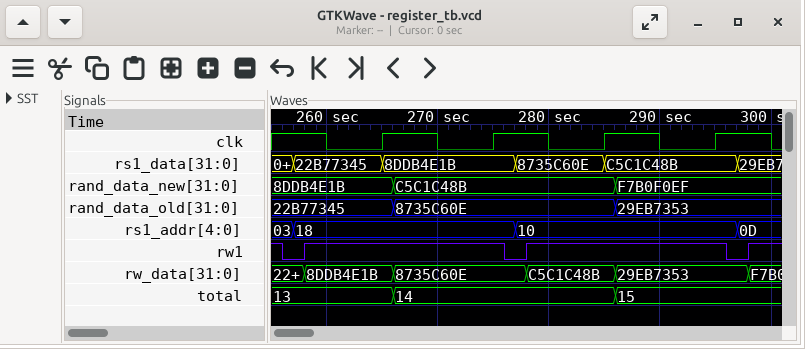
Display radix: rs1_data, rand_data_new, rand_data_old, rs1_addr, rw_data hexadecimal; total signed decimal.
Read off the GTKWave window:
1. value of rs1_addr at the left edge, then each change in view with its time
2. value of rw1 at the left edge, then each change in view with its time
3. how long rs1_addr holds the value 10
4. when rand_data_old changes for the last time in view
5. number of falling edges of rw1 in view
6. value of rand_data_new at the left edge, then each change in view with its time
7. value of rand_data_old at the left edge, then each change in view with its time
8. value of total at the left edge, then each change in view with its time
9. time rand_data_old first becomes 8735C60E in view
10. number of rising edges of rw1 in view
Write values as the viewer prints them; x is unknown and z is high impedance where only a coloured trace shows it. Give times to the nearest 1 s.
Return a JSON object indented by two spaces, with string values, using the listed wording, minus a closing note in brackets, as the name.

{
  "value of rs1_addr at the left edge, then each change in view with its time": "03, 18 at 257 s, 10 at 277 s, 0D at 297 s",
  "value of rw1 at the left edge, then each change in view with its time": "1, 0 at 256 s, 1 at 258 s, 0 at 276 s, 1 at 278 s, 0 at 296 s, 1 at 298 s",
  "how long rs1_addr holds the value 10": "20 s",
  "when rand_data_old changes for the last time in view": "286 s",
  "number of falling edges of rw1 in view": "3",
  "value of rand_data_new at the left edge, then each change in view with its time": "8DDB4E1B, C5C1C48B at 266 s, F7B0F0EF at 286 s",
  "value of rand_data_old at the left edge, then each change in view with its time": "22B77345, 8735C60E at 266 s, 29EB7353 at 286 s",
  "value of total at the left edge, then each change in view with its time": "13, 14 at 266 s, 15 at 286 s",
  "time rand_data_old first becomes 8735C60E in view": "266 s",
  "number of rising edges of rw1 in view": "3"
}
